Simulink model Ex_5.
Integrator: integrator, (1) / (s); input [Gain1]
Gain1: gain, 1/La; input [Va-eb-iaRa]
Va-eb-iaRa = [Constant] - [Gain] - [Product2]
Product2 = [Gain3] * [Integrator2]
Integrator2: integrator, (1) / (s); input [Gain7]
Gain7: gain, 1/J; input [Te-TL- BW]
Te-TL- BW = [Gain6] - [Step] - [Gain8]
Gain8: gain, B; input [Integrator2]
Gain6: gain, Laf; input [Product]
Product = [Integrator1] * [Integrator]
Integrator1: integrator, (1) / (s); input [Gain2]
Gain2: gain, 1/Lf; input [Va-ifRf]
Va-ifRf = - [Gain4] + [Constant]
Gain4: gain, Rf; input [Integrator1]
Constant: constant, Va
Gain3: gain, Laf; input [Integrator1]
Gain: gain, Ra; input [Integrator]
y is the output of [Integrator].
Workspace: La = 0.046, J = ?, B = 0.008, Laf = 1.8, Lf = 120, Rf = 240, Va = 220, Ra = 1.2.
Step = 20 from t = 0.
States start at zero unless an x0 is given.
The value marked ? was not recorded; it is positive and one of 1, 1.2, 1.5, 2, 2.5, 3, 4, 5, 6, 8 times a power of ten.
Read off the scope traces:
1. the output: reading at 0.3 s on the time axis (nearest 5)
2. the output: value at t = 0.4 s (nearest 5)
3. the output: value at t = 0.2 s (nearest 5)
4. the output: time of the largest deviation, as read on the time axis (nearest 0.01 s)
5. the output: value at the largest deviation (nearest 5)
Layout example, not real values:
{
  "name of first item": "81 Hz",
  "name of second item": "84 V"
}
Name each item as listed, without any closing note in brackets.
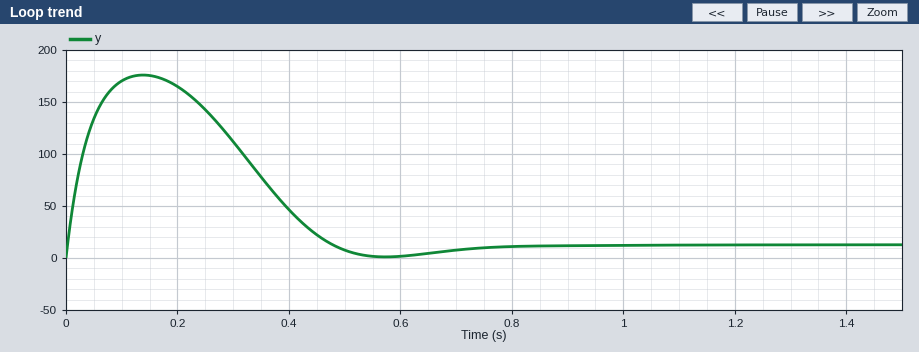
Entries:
{
  "the output: reading at 0.3 s on the time axis": "110",
  "the output: value at t = 0.4 s": "45",
  "the output: value at t = 0.2 s": "165",
  "the output: time of the largest deviation, as read on the time axis": "0.14 s",
  "the output: value at the largest deviation": "175"
}
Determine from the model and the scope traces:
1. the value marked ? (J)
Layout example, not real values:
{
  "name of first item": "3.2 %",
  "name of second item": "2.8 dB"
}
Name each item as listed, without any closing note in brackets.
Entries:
{
  "the value marked ?": "0.08"
}
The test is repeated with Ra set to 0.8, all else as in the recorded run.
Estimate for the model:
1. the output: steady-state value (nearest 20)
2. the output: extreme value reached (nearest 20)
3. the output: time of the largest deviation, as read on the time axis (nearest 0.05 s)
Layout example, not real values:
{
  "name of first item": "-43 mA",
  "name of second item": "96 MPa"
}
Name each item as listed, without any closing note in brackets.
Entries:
{
  "the output: steady-state value": "20",
  "the output: extreme value reached": "240",
  "the output: time of the largest deviation, as read on the time axis": "0.15 s"
}
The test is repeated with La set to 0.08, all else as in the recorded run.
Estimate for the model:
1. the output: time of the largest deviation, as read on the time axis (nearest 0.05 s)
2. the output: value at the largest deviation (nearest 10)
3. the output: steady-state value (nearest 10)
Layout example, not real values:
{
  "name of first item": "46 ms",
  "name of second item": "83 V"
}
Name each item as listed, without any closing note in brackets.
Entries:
{
  "the output: time of the largest deviation, as read on the time axis": "0.20 s",
  "the output: value at the largest deviation": "170",
  "the output: steady-state value": "10"
}
